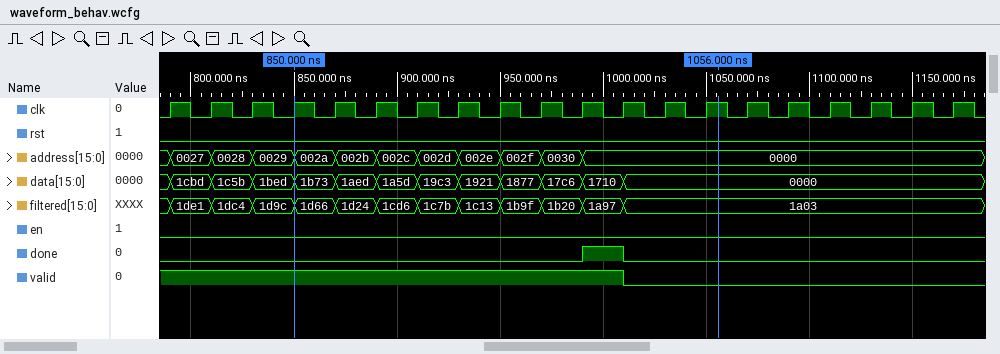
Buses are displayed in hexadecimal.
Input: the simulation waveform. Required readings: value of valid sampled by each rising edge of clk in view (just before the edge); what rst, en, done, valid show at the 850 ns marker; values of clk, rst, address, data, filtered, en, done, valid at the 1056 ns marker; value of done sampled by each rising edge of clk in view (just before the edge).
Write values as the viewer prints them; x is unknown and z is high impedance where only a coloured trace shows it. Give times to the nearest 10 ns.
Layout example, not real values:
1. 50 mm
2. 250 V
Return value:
1. 1 1 1 1 1 1 1 1 1 1 1 1 0 0 0 0 0 0 0 0
2. rst=0, en=0, done=0, valid=1
3. clk=1, rst=0, address=0000, data=0000, filtered=1a03, en=0, done=0, valid=0
4. 0 0 0 0 0 0 0 0 0 0 0 1 0 0 0 0 0 0 0 0
